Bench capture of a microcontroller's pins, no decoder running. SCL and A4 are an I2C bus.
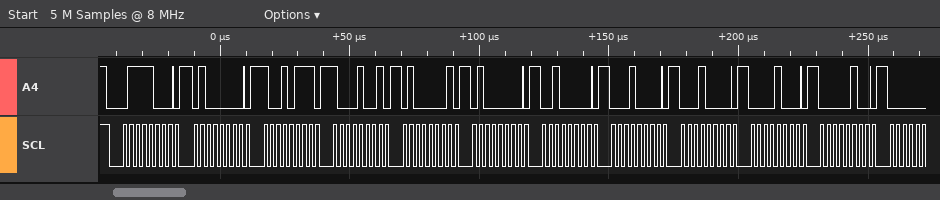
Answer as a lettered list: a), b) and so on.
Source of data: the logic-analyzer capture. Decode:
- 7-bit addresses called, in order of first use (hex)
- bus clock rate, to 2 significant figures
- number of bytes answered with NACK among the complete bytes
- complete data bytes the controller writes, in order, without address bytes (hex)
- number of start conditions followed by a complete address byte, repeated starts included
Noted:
a) 0x3C
b) 400 kHz
c) 0
d) 40 97 89 41 40 20 10 10 08 04
e) 1
